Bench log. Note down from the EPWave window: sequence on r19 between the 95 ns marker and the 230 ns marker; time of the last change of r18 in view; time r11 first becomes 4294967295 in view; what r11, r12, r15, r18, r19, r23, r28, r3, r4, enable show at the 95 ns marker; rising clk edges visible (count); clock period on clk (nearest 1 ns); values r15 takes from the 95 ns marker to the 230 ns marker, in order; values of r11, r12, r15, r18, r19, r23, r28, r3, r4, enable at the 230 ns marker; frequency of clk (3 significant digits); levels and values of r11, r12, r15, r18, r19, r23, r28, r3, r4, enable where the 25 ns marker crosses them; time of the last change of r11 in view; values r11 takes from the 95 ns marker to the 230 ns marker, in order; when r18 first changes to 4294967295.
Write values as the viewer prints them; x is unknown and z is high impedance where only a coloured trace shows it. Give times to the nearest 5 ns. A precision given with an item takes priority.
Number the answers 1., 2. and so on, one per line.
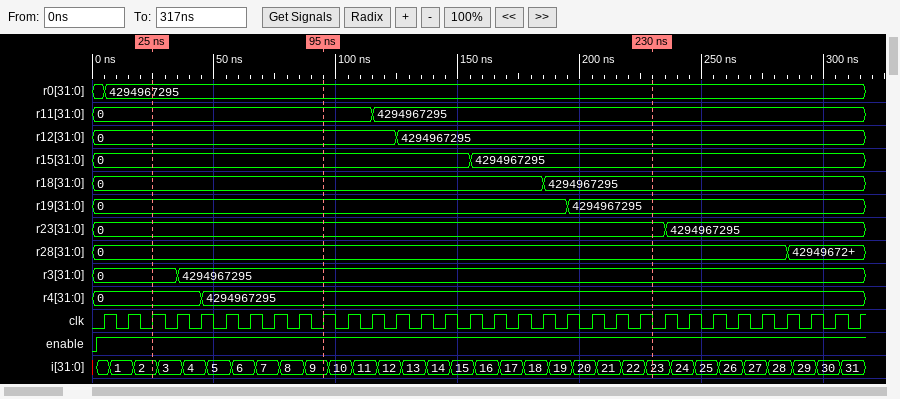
1. 0, 4294967295
2. 185 ns
3. 115 ns
4. r11=0, r12=0, r15=0, r18=0, r19=0, r23=0, r28=0, r3=4294967295, r4=4294967295, enable=1
5. 32
6. 10 ns
7. 0, 4294967295
8. r11=4294967295, r12=4294967295, r15=4294967295, r18=4294967295, r19=4294967295, r23=0, r28=0, r3=4294967295, r4=4294967295, enable=1
9. 100 MHz
10. r11=0, r12=0, r15=0, r18=0, r19=0, r23=0, r28=0, r3=0, r4=0, enable=1
11. 115 ns
12. 0, 4294967295
13. 185 ns
